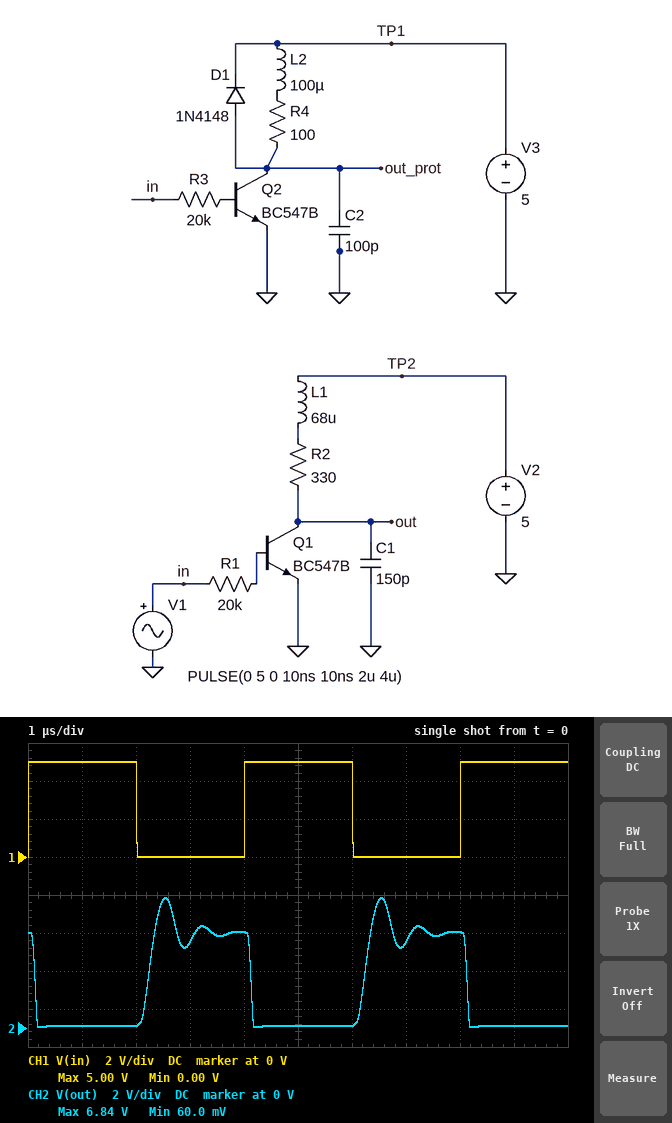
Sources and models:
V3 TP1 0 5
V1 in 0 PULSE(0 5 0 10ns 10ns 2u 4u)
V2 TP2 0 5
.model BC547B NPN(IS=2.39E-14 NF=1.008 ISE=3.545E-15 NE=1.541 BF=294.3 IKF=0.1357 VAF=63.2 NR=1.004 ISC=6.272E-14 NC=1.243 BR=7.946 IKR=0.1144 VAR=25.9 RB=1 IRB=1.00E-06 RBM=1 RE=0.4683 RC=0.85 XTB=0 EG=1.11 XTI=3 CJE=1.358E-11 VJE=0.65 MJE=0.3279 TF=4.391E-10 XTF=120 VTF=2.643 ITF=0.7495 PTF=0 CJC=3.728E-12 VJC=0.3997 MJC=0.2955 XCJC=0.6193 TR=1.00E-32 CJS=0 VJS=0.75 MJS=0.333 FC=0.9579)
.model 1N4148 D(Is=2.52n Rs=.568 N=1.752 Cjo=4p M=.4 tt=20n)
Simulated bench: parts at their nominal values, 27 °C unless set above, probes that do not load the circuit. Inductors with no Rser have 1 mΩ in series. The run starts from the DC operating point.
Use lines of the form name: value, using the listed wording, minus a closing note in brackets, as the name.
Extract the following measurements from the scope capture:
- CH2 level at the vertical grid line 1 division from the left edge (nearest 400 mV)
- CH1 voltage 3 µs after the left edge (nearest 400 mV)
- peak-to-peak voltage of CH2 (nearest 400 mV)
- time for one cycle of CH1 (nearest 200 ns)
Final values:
CH2 level at the vertical grid line 1 division from the left edge: 0 V
CH1 voltage 3 µs after the left edge: 0 V
peak-to-peak voltage of CH2: 6.8 V
time for one cycle of CH1: 4.0 µs
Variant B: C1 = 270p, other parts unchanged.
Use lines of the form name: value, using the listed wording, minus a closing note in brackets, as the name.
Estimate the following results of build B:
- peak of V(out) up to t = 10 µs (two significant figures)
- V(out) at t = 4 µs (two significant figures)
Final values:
peak of V(out) up to t = 10 µs: 6.7 V
V(out) at t = 4 µs: 4.9 V
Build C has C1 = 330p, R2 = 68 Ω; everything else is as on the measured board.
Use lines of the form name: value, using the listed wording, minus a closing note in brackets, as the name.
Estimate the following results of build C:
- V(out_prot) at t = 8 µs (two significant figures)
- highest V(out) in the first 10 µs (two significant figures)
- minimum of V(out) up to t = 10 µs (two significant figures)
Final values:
V(out_prot) at t = 8 µs: 5.6 V
highest V(out) in the first 10 µs: 15 V
minimum of V(out) up to t = 10 µs: -2.4 V
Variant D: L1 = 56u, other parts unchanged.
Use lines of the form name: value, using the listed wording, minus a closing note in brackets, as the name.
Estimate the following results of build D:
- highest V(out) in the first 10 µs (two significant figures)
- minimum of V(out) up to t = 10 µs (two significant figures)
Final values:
highest V(out) in the first 10 µs: 6.3 V
minimum of V(out) up to t = 10 µs: 65 mV
